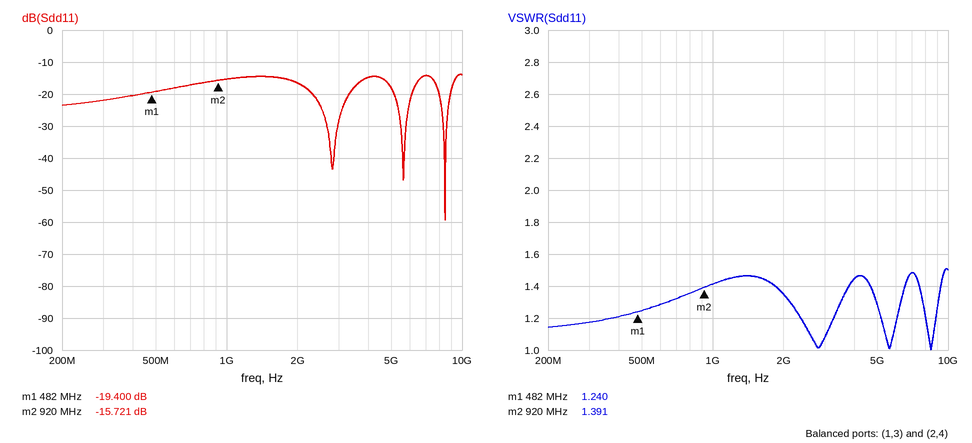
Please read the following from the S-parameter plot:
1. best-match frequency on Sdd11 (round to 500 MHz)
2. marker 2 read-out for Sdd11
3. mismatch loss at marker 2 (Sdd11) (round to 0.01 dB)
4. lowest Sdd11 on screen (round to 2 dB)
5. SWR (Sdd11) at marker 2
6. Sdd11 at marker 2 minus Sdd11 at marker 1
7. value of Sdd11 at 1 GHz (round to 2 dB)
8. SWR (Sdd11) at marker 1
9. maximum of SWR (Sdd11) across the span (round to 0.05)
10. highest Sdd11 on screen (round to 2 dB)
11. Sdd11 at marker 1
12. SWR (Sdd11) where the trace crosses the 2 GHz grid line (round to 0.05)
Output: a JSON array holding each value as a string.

["8.5 GHz", "-15.721 dB", "0.12 dB", "-60 dB", "1.391", "3.679 dB", "-16 dB", "1.240", "1.50", "-14 dB", "-19.400 dB", "1.35"]
